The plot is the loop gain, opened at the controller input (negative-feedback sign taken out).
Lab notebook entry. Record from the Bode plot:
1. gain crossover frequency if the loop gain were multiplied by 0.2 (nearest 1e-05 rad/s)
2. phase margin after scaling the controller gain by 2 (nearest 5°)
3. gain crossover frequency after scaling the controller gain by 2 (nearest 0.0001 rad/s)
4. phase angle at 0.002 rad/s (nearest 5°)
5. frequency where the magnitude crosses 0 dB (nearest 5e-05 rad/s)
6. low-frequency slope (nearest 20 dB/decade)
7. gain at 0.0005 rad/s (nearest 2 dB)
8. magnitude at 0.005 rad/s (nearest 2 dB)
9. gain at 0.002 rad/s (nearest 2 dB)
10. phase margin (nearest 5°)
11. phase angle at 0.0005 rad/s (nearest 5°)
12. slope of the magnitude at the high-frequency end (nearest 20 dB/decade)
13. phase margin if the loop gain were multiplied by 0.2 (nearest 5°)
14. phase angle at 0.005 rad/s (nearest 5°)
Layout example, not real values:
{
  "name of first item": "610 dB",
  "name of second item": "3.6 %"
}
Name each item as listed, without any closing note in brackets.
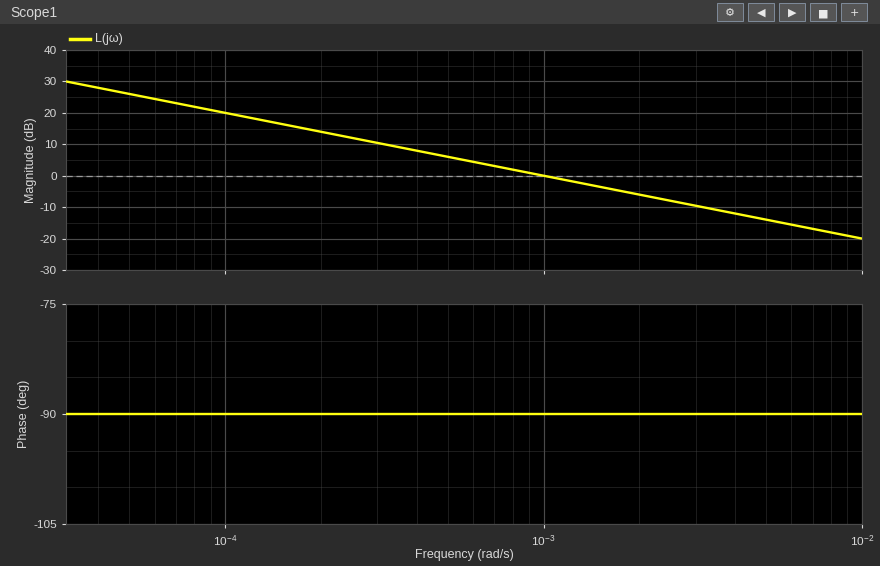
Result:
{
  "gain crossover frequency if the loop gain were multiplied by 0.2": "0.00020 rad/s",
  "phase margin after scaling the controller gain by 2": "90°",
  "gain crossover frequency after scaling the controller gain by 2": "0.0020 rad/s",
  "phase angle at 0.002 rad/s": "-90°",
  "frequency where the magnitude crosses 0 dB": "0.00100 rad/s",
  "low-frequency slope": "-20 dB/decade",
  "gain at 0.0005 rad/s": "6 dB",
  "magnitude at 0.005 rad/s": "-14 dB",
  "gain at 0.002 rad/s": "-6 dB",
  "phase margin": "90°",
  "phase angle at 0.0005 rad/s": "-90°",
  "slope of the magnitude at the high-frequency end": "-20 dB/decade",
  "phase margin if the loop gain were multiplied by 0.2": "90°",
  "phase angle at 0.005 rad/s": "-90°"
}
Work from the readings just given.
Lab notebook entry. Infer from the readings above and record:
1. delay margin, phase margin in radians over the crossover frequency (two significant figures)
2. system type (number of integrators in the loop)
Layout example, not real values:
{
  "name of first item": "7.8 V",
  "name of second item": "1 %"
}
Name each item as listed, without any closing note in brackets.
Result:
{
  "delay margin, phase margin in radians over the crossover frequency": "1600 s",
  "system type": "1"
}
